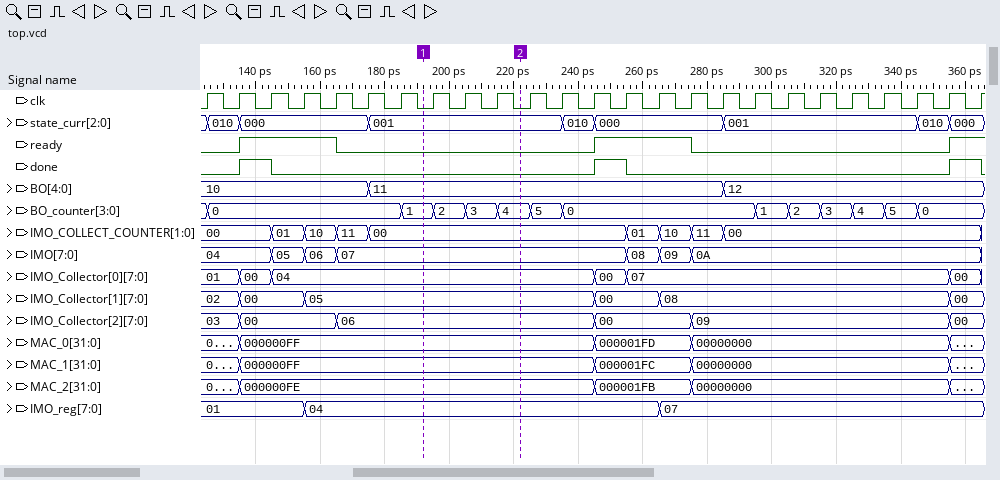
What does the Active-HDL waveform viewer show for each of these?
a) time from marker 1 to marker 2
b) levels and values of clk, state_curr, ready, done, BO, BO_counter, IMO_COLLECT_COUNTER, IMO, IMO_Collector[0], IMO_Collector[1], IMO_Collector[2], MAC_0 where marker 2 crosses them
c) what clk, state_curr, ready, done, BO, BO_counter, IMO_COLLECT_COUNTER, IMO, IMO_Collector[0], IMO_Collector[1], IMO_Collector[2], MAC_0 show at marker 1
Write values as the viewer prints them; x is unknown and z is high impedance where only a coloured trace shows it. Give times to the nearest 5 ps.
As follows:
30 ps
clk=0, state_curr=001, ready=0, done=0, BO=11, BO_counter=4, IMO_COLLECT_COUNTER=00, IMO=07, IMO_Collector[0]=04, IMO_Collector[1]=05, IMO_Collector[2]=06, MAC_0=000000FF
clk=0, state_curr=001, ready=0, done=0, BO=11, BO_counter=1, IMO_COLLECT_COUNTER=00, IMO=07, IMO_Collector[0]=04, IMO_Collector[1]=05, IMO_Collector[2]=06, MAC_0=000000FF
